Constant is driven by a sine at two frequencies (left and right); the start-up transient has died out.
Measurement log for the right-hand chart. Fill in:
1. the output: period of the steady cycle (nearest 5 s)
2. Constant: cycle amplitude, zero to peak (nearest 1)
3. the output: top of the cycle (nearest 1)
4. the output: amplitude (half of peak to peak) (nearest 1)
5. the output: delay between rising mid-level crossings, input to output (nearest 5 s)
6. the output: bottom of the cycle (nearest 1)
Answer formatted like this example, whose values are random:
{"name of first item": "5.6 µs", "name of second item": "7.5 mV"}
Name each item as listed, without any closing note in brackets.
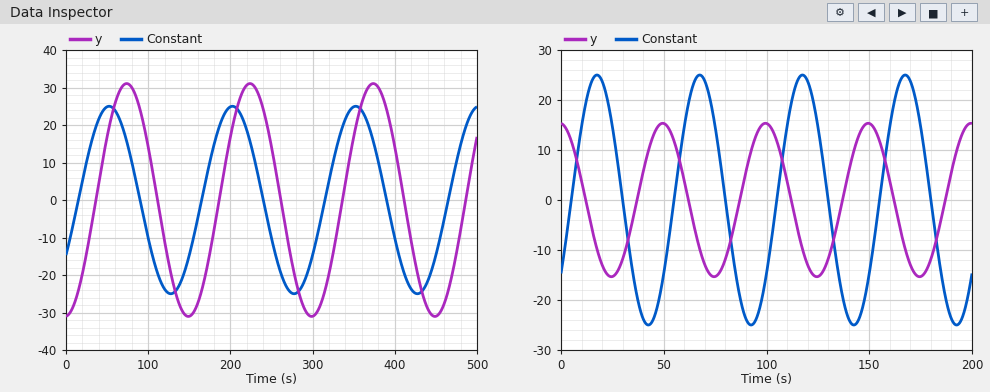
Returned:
{"the output: period of the steady cycle": "50 s", "Constant: cycle amplitude, zero to peak": "25", "the output: top of the cycle": "15", "the output: amplitude (half of peak to peak)": "15", "the output: delay between rising mid-level crossings, input to output": "30 s", "the output: bottom of the cycle": "-15"}
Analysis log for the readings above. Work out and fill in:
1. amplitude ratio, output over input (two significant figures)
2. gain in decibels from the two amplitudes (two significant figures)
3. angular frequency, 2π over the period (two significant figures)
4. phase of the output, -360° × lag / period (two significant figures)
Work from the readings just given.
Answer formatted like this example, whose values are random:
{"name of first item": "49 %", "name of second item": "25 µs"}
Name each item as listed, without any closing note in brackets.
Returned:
{"amplitude ratio, output over input": "0.60", "gain in decibels from the two amplitudes": "-4.4 dB", "angular frequency, 2π over the period": "0.13 rad/s", "phase of the output, -360° × lag / period": "-220°"}
